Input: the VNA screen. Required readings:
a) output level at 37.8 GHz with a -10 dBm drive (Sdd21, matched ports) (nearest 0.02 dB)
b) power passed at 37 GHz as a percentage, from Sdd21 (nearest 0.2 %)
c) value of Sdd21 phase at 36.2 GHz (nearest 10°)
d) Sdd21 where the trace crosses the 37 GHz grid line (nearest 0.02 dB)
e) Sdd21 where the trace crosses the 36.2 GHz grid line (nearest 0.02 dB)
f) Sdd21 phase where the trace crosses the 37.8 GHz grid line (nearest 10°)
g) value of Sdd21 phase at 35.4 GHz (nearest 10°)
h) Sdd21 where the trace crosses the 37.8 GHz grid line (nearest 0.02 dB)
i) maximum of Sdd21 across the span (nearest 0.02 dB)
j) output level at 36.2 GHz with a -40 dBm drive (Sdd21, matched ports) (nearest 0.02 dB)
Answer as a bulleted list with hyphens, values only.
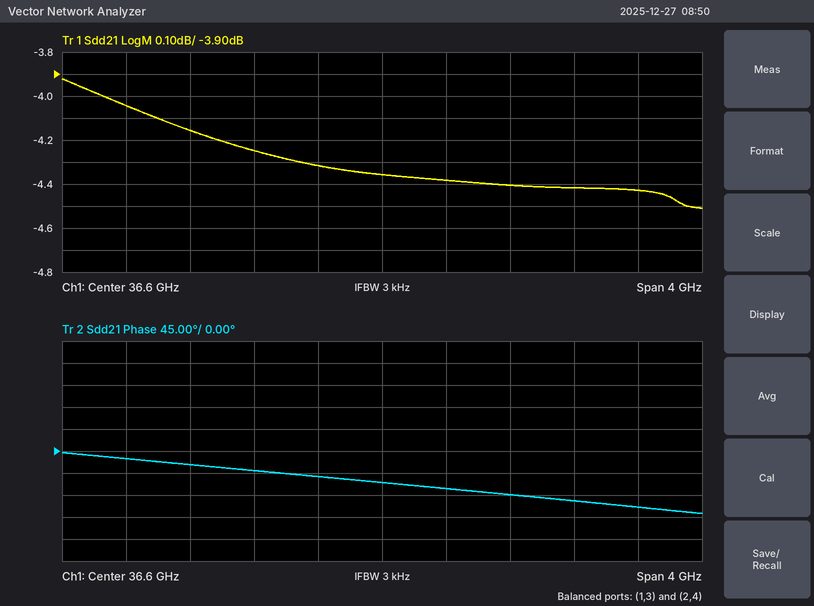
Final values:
- -14.42 dBm
- 36.4 %
- -50°
- -4.38 dB
- -4.32 dB
- -100°
- -30°
- -4.42 dB
- -3.92 dB
- -44.32 dBm
